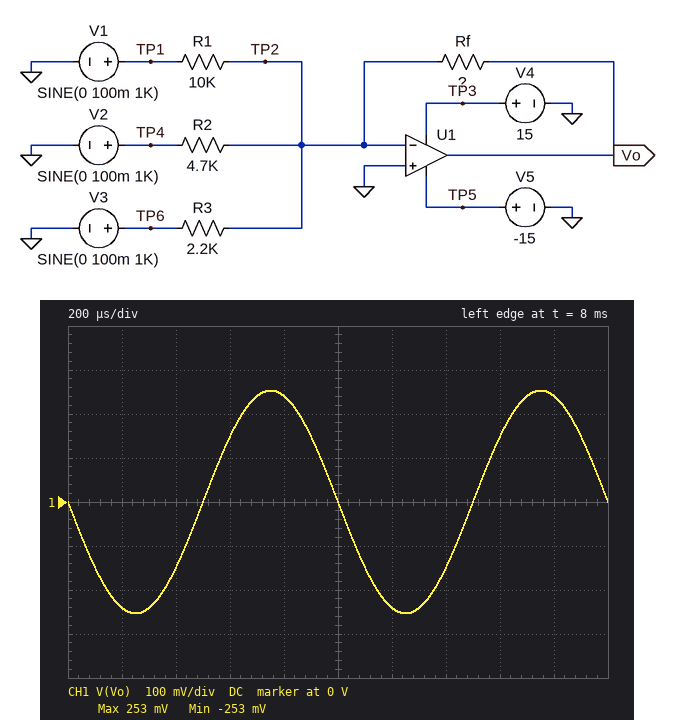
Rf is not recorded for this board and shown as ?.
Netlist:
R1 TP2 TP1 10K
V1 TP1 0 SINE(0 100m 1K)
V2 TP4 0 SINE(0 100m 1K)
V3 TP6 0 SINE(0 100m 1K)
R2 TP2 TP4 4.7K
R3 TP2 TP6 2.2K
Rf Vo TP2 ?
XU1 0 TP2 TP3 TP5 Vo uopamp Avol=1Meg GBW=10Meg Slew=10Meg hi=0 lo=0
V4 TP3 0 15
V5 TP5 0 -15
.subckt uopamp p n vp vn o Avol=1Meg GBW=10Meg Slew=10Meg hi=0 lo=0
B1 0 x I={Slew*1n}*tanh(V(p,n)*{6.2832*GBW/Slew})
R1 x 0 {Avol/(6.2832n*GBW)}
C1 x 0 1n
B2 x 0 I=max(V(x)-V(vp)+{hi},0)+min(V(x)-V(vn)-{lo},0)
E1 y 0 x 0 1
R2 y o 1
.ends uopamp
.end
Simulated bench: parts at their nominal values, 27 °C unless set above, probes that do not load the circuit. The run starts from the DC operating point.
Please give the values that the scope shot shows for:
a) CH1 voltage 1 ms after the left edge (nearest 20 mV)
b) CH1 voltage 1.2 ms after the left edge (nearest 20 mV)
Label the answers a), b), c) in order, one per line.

a) 0 V
b) -240 mV
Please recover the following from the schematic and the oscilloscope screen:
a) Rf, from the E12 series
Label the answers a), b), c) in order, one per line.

a) 3.3 kΩ
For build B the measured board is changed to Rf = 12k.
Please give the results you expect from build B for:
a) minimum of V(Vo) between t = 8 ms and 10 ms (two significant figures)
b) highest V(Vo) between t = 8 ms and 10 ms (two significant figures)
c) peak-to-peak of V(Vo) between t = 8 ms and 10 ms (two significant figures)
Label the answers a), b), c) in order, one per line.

a) -920 mV
b) 920 mV
c) 1.8 V
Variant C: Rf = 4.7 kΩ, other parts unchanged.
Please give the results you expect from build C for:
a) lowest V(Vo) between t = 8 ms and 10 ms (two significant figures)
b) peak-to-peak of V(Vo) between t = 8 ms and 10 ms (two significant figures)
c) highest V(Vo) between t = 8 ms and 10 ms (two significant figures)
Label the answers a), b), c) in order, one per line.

a) -360 mV
b) 720 mV
c) 360 mV
